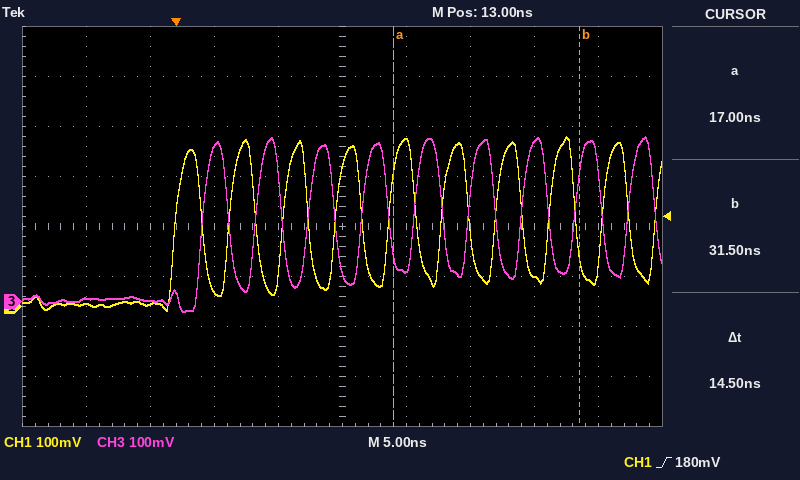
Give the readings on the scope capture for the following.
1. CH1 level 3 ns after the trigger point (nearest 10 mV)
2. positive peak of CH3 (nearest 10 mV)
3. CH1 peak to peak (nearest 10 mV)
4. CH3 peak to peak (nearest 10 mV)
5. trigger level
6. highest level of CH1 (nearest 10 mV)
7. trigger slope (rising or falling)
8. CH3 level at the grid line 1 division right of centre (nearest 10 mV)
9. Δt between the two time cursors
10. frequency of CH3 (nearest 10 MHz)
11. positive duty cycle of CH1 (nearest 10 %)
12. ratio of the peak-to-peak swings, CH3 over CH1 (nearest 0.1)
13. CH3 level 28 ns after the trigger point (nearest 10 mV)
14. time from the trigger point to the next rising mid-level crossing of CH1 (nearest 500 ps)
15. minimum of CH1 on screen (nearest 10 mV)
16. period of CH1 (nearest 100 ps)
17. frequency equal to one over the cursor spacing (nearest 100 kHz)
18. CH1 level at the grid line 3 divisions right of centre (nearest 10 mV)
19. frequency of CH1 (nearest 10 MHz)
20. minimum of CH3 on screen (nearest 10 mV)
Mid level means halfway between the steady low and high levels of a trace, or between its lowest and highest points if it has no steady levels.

30 mV
330 mV
350 mV
350 mV
180 mV
340 mV
rising
70 mV
14.5 ns
240 MHz
50 %
1.0
320 mV
4.0 ns
-10 mV
4.2 ns
69.0 MHz
60 mV
240 MHz
-20 mV
